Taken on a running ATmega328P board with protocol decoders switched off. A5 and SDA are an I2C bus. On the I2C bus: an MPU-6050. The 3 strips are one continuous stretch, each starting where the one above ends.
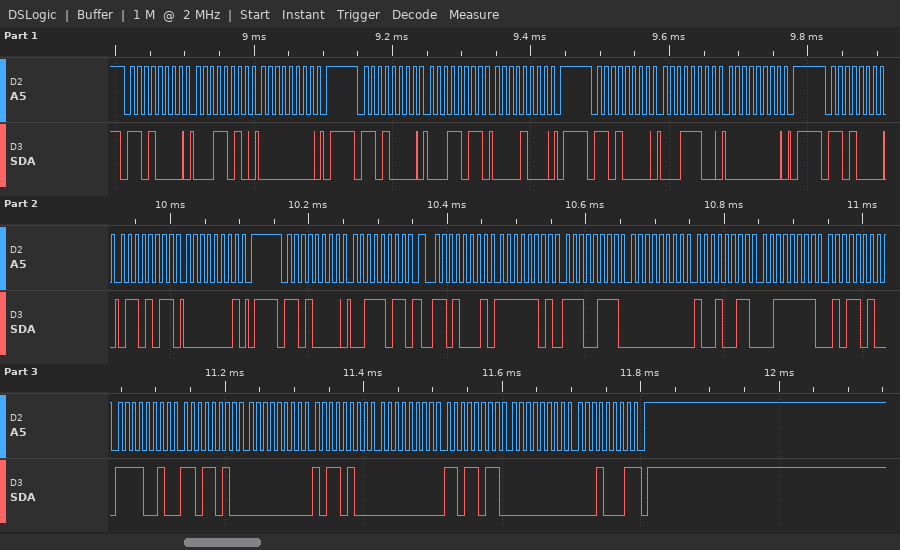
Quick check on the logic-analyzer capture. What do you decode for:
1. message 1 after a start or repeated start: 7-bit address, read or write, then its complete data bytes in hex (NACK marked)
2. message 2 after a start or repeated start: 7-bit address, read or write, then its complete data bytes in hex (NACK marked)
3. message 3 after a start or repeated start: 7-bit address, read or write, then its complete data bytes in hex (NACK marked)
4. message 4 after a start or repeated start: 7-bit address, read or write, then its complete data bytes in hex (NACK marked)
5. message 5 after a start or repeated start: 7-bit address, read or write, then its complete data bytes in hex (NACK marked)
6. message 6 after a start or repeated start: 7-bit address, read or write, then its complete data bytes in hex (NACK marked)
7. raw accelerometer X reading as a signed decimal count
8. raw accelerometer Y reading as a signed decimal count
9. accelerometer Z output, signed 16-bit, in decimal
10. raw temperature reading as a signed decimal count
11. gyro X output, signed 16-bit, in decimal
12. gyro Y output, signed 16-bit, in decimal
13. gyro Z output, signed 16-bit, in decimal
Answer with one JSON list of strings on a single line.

["0x68 write: 1A 00", "0x68 write: 1B 08", "0x68 write: 1C 00", "0x68 write: 6B 01", "0x68 write: 3B", "0x68 read: FD E7 00 93 3F 5A F2 DA 00 B4 00 DB 00 11 NACK", "-537", "147", "16218", "-3366", "180", "219", "17"]
